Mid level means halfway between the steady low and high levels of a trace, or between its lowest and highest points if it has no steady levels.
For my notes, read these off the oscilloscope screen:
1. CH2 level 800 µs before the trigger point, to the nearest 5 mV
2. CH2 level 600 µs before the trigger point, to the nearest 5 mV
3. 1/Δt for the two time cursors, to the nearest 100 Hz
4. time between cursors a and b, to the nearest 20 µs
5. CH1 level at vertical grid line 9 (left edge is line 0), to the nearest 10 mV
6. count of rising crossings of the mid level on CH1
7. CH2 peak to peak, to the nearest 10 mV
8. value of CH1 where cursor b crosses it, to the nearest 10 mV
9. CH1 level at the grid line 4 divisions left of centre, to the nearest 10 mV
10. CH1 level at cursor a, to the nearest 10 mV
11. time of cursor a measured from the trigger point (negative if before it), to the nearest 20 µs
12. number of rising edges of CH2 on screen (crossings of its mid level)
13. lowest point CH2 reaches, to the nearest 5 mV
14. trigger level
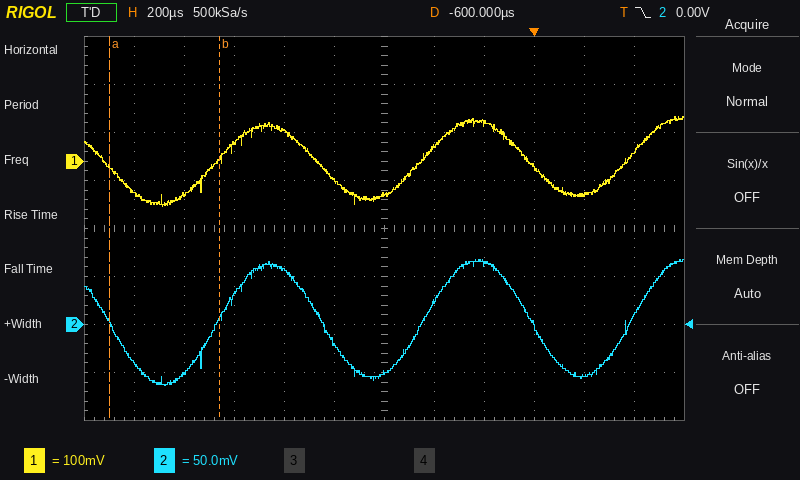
-20 mV
-50 mV
2.3 kHz
440 µs
-10 mV
3
130 mV
10 mV
-70 mV
-10 mV
-1.70 ms
3
-65 mV
0.00 V
